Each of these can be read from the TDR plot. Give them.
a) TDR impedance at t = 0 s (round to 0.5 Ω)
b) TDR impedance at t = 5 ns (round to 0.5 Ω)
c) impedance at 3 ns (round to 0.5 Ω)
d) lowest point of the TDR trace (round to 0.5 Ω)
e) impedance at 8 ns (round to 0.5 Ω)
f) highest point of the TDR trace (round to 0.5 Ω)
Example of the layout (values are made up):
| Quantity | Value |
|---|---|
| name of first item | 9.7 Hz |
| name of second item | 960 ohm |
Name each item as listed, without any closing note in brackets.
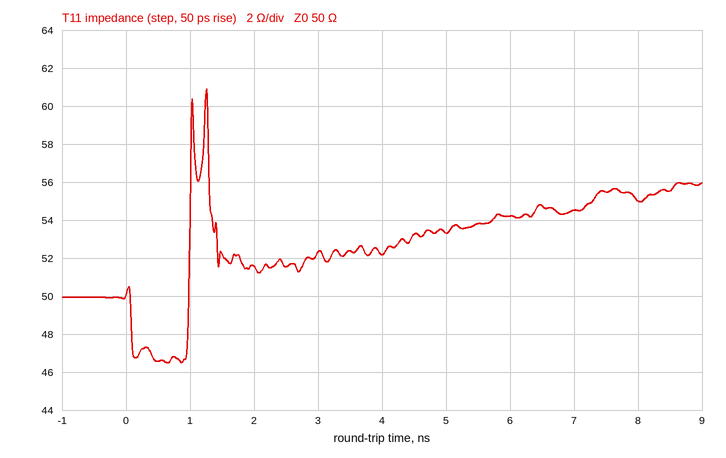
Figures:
| Quantity | Value |
|---|---|
| TDR impedance at t = 0 s | 50.0 Ω |
| TDR impedance at t = 5 ns | 53.5 Ω |
| impedance at 3 ns | 52.5 Ω |
| lowest point of the TDR trace | 46.5 Ω |
| impedance at 8 ns | 55.0 Ω |
| highest point of the TDR trace | 61.0 Ω |
